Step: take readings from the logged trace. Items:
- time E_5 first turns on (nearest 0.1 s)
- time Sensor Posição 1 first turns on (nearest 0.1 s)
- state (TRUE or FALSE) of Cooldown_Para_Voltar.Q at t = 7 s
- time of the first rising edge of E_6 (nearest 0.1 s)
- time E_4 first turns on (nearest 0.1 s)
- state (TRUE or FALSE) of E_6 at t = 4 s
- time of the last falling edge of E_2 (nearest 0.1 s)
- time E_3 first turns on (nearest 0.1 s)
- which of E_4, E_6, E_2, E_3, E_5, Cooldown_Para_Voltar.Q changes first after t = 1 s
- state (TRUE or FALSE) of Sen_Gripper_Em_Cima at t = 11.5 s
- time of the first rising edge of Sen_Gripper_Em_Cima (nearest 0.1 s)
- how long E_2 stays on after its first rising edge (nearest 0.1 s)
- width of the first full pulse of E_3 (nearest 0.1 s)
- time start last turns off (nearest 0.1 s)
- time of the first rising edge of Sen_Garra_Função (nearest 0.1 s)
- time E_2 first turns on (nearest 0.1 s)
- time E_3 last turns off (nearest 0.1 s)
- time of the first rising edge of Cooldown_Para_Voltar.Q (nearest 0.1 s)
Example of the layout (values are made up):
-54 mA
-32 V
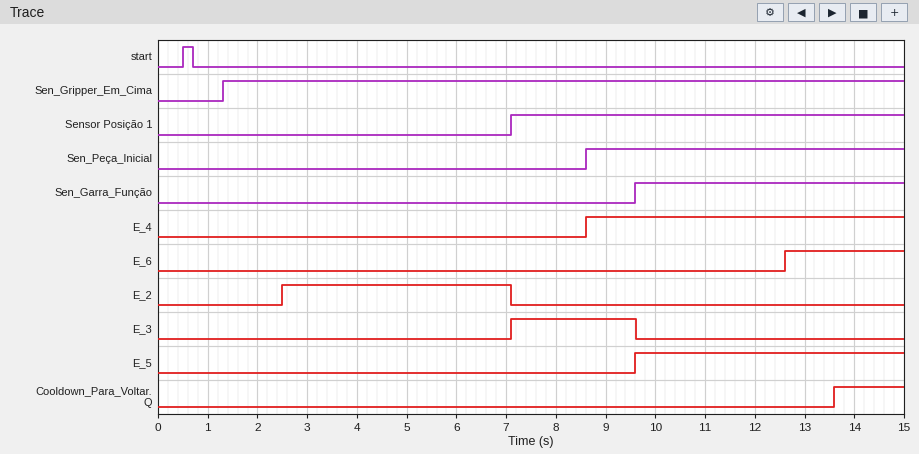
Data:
9.6 s
7.1 s
FALSE
12.6 s
8.6 s
FALSE
7.1 s
7.1 s
E_2
TRUE
1.3 s
4.6 s
2.5 s
0.7 s
9.6 s
2.5 s
9.6 s
13.6 s
